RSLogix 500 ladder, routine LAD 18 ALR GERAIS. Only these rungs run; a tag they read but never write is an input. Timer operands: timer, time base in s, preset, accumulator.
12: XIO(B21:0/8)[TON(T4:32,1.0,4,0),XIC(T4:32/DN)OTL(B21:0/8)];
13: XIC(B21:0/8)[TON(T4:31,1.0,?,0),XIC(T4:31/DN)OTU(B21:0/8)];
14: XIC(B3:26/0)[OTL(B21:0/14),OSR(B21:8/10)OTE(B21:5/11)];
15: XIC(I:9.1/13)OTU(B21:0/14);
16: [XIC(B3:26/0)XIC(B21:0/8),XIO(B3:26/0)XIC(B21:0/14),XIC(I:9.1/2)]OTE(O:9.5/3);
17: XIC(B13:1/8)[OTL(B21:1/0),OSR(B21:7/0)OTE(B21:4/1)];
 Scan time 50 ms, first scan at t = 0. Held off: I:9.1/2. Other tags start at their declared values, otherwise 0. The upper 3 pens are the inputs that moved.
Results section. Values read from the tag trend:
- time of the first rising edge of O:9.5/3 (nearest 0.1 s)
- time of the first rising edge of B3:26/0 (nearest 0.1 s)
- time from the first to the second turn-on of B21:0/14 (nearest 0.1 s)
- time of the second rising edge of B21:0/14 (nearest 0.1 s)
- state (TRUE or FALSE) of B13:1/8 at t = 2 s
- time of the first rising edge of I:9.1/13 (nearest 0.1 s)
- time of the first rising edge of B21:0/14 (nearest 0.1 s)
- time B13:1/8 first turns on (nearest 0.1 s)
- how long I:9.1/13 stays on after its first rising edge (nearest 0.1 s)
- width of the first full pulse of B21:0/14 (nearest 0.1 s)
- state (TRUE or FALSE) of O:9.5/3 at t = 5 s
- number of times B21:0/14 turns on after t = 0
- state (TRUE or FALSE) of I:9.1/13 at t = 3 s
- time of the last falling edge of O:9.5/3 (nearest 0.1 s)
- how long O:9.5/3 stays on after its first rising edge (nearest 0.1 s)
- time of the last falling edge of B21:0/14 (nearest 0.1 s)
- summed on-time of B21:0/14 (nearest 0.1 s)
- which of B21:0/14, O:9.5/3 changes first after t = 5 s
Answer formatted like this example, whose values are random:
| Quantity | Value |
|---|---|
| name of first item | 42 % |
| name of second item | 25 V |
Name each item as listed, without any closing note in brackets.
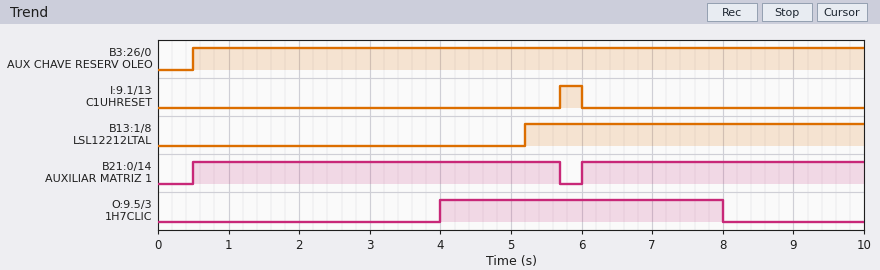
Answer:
| Quantity | Value |
|---|---|
| time of the first rising edge of O:9.5/3 | 4.0 s |
| time of the first rising edge of B3:26/0 | 0.5 s |
| time from the first to the second turn-on of B21:0/14 | 5.5 s |
| time of the second rising edge of B21:0/14 | 6.0 s |
| state (TRUE or FALSE) of B13:1/8 at t = 2 s | FALSE |
| time of the first rising edge of I:9.1/13 | 5.7 s |
| time of the first rising edge of B21:0/14 | 0.5 s |
| time B13:1/8 first turns on | 5.2 s |
| how long I:9.1/13 stays on after its first rising edge | 0.3 s |
| width of the first full pulse of B21:0/14 | 5.2 s |
| state (TRUE or FALSE) of O:9.5/3 at t = 5 s | TRUE |
| number of times B21:0/14 turns on after t = 0 | 2 |
| state (TRUE or FALSE) of I:9.1/13 at t = 3 s | FALSE |
| time of the last falling edge of O:9.5/3 | 8.0 s |
| how long O:9.5/3 stays on after its first rising edge | 4.0 s |
| time of the last falling edge of B21:0/14 | 5.7 s |
| summed on-time of B21:0/14 | 9.2 s |
| which of B21:0/14, O:9.5/3 changes first after t = 5 s | B21:0/14 |
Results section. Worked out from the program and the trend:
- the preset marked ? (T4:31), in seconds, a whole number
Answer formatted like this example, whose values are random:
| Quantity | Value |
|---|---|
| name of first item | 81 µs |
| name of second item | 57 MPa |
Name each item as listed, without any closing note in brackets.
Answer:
| Quantity | Value |
|---|---|
| the preset marked ? (T4:31), in seconds, a whole number | 4 s |
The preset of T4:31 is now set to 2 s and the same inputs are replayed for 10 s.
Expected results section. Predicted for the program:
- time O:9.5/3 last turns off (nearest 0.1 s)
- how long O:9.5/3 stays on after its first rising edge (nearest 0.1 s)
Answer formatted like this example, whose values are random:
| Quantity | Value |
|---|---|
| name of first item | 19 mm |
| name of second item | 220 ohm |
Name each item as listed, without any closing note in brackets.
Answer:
| Quantity | Value |
|---|---|
| time O:9.5/3 last turns off | 6.0 s |
| how long O:9.5/3 stays on after its first rising edge | 2.0 s |
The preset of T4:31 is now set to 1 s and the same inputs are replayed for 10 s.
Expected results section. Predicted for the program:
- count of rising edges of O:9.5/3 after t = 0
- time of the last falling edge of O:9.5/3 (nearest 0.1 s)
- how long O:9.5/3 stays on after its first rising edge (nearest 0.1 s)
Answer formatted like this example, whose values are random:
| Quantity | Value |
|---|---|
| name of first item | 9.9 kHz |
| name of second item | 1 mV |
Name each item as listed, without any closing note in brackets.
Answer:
| Quantity | Value |
|---|---|
| count of rising edges of O:9.5/3 after t = 0 | 2 |
| time of the last falling edge of O:9.5/3 | 5.0 s |
| how long O:9.5/3 stays on after its first rising edge | 1.0 s |
